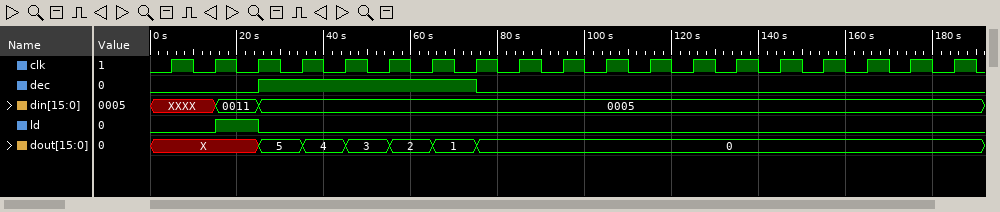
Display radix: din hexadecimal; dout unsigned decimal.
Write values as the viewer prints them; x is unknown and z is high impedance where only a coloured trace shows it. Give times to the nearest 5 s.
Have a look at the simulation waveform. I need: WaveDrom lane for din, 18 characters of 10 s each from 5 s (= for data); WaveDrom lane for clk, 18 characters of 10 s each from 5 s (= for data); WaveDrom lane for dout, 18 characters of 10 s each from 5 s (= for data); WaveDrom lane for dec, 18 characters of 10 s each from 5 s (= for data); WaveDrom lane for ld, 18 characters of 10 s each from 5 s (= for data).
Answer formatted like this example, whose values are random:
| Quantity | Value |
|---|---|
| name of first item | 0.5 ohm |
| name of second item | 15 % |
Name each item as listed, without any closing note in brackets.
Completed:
| Quantity | Value |
|---|---|
| WaveDrom lane for din, 18 characters of 10 s each from 5 s | {name: 'din', wave: 'x==...............', data: '0011 0005'} |
| WaveDrom lane for clk, 18 characters of 10 s each from 5 s | {name: 'clk', wave: 'p.................'} |
| WaveDrom lane for dout, 18 characters of 10 s each from 5 s | {name: 'dout', wave: 'x.======..........', data: '5 4 3 2 1 0'} |
| WaveDrom lane for dec, 18 characters of 10 s each from 5 s | {name: 'dec', wave: '0.1....0..........'} |
| WaveDrom lane for ld, 18 characters of 10 s each from 5 s | {name: 'ld', wave: '010...............'} |
